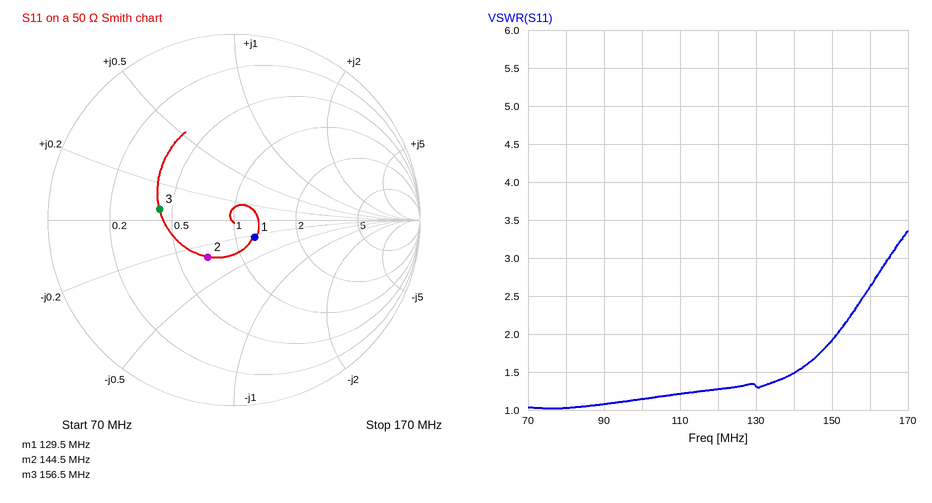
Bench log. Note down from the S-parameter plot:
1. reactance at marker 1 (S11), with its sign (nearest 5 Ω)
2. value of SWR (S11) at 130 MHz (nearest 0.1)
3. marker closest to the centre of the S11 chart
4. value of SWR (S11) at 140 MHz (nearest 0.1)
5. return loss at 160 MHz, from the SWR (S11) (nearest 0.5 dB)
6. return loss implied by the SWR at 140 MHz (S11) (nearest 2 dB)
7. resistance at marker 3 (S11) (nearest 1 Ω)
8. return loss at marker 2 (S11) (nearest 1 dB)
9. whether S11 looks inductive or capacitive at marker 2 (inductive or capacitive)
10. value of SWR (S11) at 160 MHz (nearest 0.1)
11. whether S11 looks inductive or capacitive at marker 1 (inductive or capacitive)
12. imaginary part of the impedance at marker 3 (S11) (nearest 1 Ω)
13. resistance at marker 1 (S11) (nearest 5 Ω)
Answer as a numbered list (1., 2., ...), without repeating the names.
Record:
1. -10 Ω
2. 1.3
3. marker 1
4. 1.5
5. 7.0 dB
6. 14 dB
7. 21 Ω
8. 12 dB
9. capacitive
10. 2.6
11. capacitive
12. +3 Ω
13. 60 Ω
